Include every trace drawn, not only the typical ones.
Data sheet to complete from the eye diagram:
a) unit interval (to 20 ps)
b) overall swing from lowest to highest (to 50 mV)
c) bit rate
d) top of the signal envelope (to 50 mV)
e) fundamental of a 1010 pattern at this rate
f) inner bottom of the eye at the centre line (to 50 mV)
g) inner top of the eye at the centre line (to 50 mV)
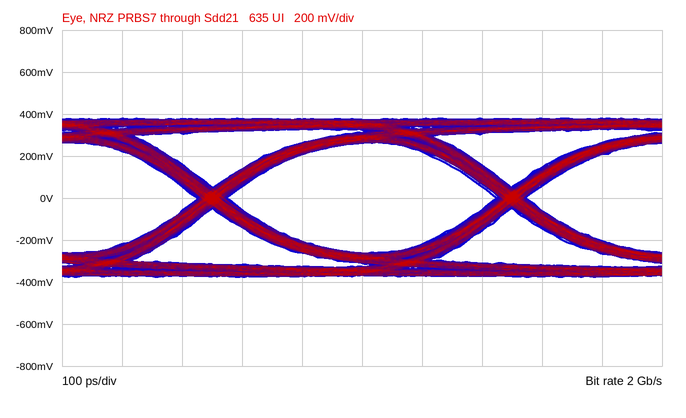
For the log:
500 ps
750 mV
2 Gb/s
400 mV
1 GHz
-250 mV
250 mV
